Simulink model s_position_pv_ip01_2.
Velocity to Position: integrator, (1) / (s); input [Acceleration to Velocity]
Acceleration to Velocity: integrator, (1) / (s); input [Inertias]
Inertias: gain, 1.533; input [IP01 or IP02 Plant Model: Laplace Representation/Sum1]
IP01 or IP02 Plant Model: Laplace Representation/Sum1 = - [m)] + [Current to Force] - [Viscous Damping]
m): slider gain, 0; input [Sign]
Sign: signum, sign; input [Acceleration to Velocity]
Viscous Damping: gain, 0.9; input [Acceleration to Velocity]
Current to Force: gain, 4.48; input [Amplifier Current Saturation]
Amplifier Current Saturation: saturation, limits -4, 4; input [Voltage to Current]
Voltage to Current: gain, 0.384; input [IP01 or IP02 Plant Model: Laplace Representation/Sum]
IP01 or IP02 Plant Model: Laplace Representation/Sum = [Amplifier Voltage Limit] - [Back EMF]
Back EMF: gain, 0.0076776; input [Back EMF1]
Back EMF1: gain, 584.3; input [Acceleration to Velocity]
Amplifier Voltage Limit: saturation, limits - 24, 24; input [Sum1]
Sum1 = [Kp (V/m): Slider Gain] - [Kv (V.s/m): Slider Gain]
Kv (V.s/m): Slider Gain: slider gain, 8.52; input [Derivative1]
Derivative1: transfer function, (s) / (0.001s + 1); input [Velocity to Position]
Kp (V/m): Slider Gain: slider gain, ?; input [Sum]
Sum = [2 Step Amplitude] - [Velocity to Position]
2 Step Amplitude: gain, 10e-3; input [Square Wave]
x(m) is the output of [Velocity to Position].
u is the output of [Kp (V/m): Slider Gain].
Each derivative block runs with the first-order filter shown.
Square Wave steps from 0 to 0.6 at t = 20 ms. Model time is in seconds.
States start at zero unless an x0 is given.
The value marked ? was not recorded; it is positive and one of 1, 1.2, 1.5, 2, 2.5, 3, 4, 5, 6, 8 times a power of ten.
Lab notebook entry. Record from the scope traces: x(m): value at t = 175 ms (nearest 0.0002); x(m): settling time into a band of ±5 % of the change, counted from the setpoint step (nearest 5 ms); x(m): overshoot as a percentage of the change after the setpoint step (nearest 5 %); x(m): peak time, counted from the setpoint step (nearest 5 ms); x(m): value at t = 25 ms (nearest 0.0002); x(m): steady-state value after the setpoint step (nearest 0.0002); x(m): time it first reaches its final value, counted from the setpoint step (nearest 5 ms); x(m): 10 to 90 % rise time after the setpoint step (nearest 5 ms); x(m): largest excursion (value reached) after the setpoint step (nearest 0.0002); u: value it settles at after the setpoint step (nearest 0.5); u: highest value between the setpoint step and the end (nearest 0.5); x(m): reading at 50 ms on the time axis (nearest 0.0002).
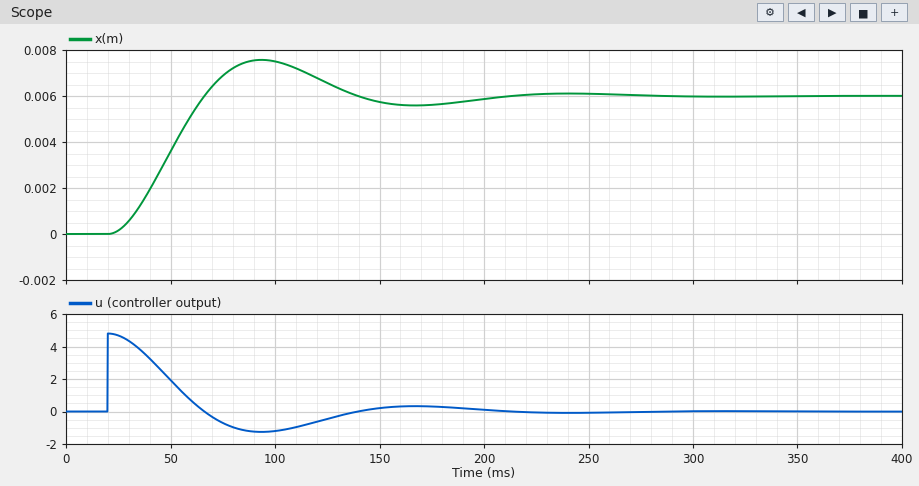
0.0056
165 ms
25 %
75 ms
0.0002
0.0060
45 ms
30 ms
0.0076
0.0
5.0
0.0036
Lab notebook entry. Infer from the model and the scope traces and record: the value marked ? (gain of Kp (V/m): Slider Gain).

800
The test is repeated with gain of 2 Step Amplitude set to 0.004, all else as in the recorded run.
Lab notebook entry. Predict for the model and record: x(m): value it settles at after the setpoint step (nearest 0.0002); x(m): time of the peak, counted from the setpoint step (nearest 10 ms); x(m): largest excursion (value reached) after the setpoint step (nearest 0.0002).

0.0024
70 ms
0.0030
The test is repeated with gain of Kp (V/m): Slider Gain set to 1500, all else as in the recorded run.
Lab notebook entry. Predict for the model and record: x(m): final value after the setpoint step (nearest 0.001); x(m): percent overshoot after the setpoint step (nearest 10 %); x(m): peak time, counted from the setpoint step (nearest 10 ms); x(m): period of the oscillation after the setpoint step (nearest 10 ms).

0.006
40 %
50 ms
100 ms
